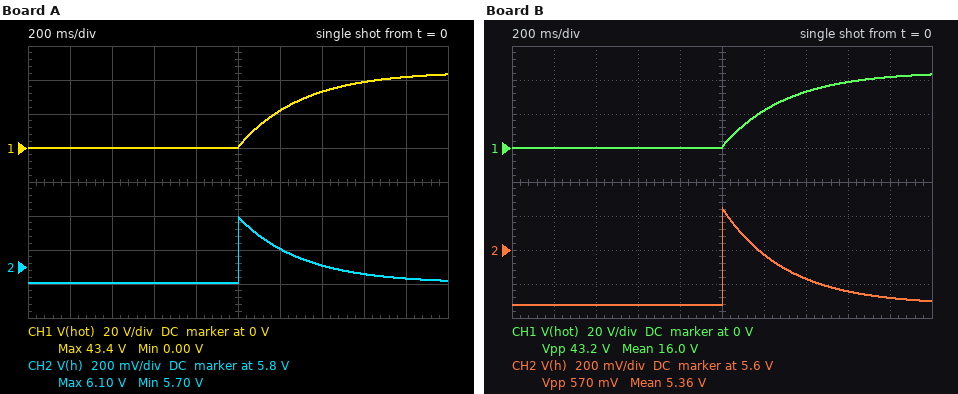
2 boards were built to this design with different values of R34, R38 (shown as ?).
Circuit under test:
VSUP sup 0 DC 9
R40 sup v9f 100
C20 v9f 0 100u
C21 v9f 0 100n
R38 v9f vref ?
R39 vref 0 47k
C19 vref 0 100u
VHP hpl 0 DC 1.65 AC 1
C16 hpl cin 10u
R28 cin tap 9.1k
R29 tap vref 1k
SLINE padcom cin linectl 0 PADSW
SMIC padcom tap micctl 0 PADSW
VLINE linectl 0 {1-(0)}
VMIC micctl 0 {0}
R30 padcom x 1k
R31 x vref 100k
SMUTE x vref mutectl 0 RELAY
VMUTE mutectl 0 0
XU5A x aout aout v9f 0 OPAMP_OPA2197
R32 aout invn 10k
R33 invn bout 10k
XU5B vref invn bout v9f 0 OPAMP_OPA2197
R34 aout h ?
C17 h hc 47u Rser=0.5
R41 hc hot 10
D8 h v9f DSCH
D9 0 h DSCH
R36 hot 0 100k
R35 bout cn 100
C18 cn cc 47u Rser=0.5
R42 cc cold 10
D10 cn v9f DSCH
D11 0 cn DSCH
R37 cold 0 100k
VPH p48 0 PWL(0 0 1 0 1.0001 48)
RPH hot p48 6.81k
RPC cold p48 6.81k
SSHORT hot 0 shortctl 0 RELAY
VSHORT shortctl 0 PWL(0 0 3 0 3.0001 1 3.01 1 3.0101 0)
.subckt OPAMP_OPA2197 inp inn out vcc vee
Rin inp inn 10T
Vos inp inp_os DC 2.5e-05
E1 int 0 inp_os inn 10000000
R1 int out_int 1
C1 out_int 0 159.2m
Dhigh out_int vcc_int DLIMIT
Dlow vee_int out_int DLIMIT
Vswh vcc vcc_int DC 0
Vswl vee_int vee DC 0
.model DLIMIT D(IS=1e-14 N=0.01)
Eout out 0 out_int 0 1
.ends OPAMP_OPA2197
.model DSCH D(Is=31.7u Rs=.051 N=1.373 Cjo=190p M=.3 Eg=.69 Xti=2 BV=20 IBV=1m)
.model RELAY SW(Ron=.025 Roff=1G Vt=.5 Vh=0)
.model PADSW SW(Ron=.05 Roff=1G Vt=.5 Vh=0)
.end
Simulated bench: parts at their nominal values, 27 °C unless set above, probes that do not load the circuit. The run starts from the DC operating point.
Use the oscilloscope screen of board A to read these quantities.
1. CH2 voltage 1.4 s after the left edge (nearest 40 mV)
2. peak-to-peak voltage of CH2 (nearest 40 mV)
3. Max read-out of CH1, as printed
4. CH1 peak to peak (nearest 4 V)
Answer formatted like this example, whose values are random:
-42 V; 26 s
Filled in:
5.80 V; 400 mV; 43.4 V; 44 V
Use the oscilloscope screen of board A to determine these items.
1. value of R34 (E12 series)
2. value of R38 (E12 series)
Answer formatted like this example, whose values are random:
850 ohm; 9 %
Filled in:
56 Ω; 27 kΩ
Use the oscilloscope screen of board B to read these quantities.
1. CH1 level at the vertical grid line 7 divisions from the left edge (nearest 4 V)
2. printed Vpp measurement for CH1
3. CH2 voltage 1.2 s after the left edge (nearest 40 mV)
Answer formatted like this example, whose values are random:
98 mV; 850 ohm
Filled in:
32 V; 43.2 V; 5.56 V
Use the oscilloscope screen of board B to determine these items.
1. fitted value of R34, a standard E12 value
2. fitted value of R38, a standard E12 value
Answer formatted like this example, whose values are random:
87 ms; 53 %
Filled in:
82 Ω; 33 kΩ
